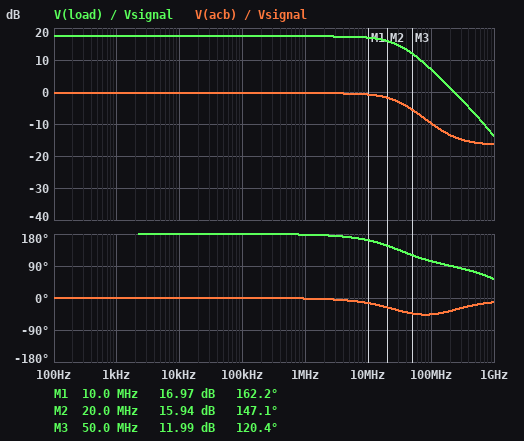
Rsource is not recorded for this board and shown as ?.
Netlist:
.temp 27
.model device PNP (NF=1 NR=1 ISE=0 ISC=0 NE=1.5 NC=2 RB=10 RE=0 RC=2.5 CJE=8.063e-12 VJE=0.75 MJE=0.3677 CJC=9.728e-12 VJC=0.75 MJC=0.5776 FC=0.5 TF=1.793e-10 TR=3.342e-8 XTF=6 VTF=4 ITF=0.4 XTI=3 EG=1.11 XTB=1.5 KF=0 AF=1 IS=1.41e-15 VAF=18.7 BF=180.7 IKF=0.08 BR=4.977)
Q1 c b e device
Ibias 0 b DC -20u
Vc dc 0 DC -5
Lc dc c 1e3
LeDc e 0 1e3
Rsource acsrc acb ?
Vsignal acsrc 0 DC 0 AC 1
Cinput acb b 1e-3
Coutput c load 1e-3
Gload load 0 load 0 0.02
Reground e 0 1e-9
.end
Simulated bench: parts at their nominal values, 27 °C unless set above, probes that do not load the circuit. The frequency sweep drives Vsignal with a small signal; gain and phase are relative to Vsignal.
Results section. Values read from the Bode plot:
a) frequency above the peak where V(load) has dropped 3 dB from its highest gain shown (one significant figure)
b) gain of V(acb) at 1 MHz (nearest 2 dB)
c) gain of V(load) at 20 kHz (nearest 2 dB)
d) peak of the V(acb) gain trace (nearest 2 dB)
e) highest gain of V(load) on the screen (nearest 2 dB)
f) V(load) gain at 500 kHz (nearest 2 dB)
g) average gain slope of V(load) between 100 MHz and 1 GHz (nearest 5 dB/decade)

30 MHz
0 dB
18 dB
0 dB
18 dB
18 dB
-20 dB/decade
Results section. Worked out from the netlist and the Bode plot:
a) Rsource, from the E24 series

62 Ω
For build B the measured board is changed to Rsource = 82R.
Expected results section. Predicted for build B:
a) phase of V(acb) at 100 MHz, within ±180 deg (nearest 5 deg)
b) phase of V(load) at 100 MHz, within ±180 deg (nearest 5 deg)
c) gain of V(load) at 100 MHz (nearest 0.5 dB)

-50 deg
100 deg
5.0 dB
